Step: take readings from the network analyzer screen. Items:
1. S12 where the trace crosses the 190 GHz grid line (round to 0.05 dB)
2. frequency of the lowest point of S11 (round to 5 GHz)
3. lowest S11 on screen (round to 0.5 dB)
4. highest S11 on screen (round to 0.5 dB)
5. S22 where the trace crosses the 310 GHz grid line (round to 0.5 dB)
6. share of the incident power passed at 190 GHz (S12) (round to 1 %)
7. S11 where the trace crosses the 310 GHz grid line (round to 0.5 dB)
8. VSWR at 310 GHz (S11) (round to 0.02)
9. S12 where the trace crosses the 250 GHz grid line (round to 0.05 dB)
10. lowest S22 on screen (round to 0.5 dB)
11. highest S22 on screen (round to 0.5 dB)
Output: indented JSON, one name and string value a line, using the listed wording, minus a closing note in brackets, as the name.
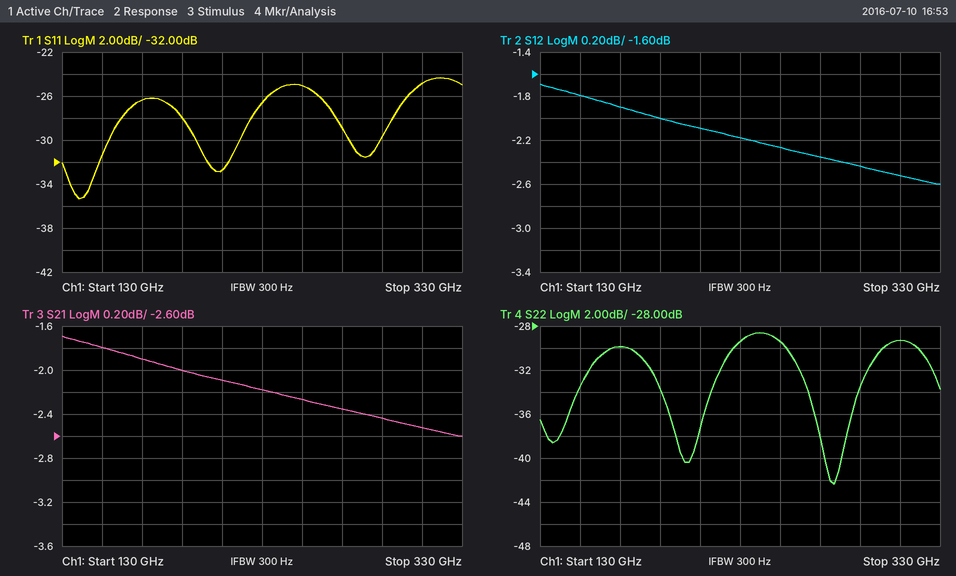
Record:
{
  "S12 where the trace crosses the 190 GHz grid line": "-2.00 dB",
  "frequency of the lowest point of S11": "140 GHz",
  "lowest S11 on screen": "-35.5 dB",
  "highest S11 on screen": "-24.5 dB",
  "S22 where the trace crosses the 310 GHz grid line": "-29.5 dB",
  "share of the incident power passed at 190 GHz (S12)": "63 %",
  "S11 where the trace crosses the 310 GHz grid line": "-25.0 dB",
  "VSWR at 310 GHz (S11)": "1.12",
  "S12 where the trace crosses the 250 GHz grid line": "-2.25 dB",
  "lowest S22 on screen": "-42.5 dB",
  "highest S22 on screen": "-28.5 dB"
}
